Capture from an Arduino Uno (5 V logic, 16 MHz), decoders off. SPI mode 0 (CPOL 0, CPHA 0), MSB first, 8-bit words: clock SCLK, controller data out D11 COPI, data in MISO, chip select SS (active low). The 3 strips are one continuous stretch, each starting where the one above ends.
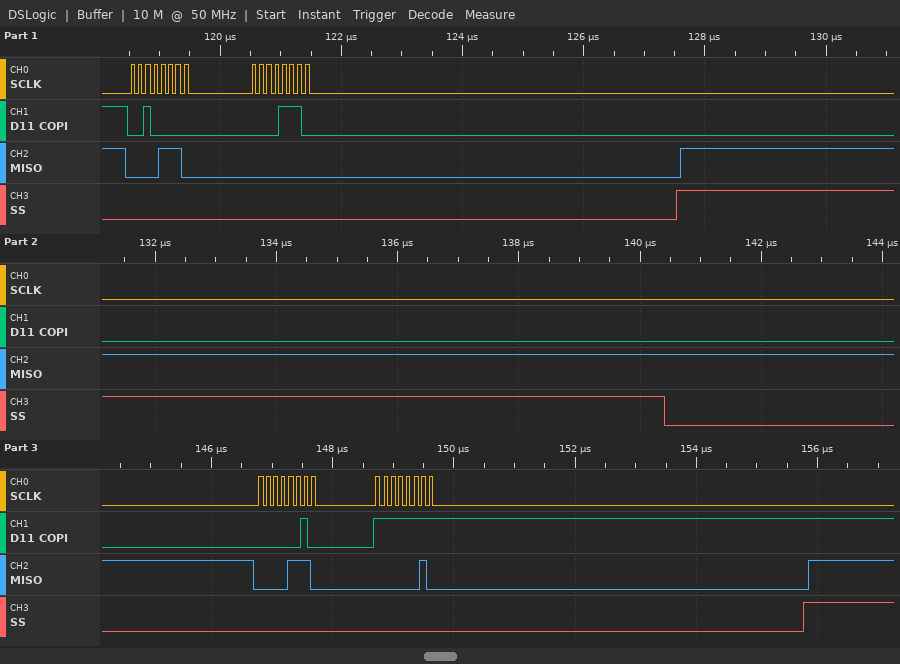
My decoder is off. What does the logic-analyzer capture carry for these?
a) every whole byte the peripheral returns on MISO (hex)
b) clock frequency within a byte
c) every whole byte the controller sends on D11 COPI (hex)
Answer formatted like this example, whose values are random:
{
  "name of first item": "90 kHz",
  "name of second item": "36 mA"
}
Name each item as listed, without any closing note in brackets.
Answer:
{
  "every whole byte the peripheral returns on MISO": "0E 00 0E 02",
  "clock frequency within a byte": "8 MHz",
  "every whole byte the controller sends on D11 COPI": "20 0E 02 FF"
}
